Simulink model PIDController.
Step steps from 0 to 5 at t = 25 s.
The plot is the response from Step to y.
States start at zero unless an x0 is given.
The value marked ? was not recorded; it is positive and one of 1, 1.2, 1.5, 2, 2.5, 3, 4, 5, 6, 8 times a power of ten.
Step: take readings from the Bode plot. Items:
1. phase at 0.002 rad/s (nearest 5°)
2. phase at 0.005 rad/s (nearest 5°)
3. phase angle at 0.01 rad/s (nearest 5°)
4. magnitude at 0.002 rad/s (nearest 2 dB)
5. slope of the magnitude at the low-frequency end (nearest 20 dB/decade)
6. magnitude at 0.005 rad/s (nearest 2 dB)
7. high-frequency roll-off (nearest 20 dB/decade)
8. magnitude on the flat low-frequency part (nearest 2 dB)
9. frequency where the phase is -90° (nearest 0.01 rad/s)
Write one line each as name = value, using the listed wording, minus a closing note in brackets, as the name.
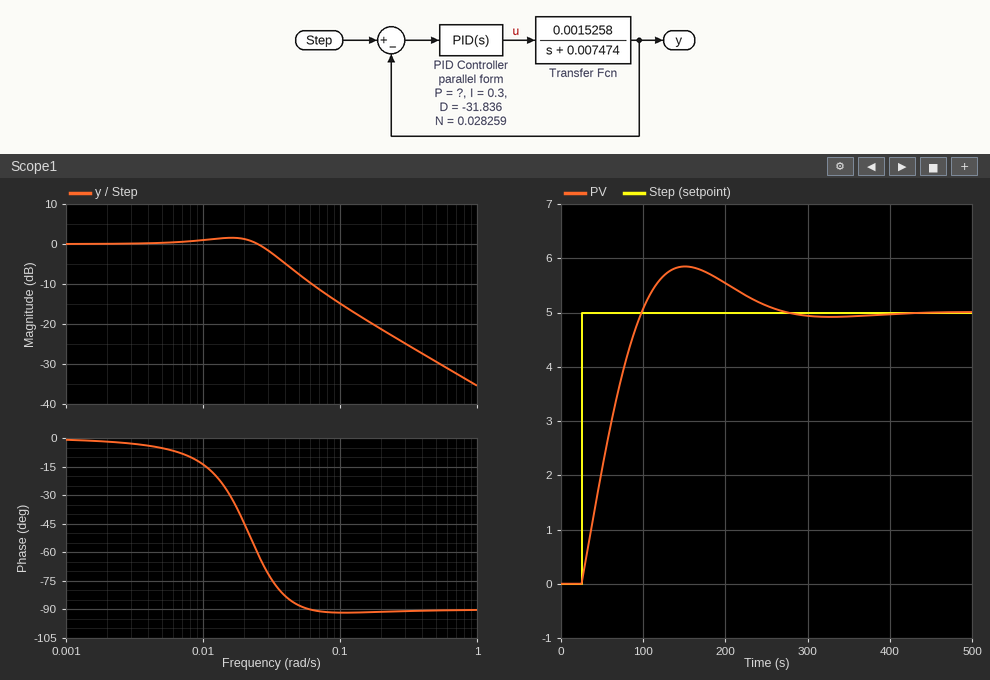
phase at 0.002 rad/s = 0°
phase at 0.005 rad/s = -5°
phase angle at 0.01 rad/s = -15°
magnitude at 0.002 rad/s = 0 dB
slope of the magnitude at the low-frequency end = 0 dB/decade
magnitude at 0.005 rad/s = 0 dB
high-frequency roll-off = -20 dB/decade
magnitude on the flat low-frequency part = 0 dB
frequency where the phase is -90° = 0.06 rad/s
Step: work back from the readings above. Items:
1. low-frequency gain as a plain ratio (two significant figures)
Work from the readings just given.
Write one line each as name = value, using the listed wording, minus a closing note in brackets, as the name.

low-frequency gain as a plain ratio = 1.0
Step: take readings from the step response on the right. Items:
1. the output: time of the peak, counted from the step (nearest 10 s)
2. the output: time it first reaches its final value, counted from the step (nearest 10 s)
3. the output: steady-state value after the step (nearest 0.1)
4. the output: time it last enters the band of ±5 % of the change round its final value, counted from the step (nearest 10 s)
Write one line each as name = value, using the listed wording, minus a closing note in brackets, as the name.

the output: time of the peak, counted from the step = 130 s
the output: time it first reaches its final value, counted from the step = 70 s
the output: steady-state value after the step = 5.0
the output: time it last enters the band of ±5 % of the change round its final value, counted from the step = 210 s
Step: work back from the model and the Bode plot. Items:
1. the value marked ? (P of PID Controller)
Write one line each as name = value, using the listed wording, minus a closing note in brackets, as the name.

the value marked ? = 12
